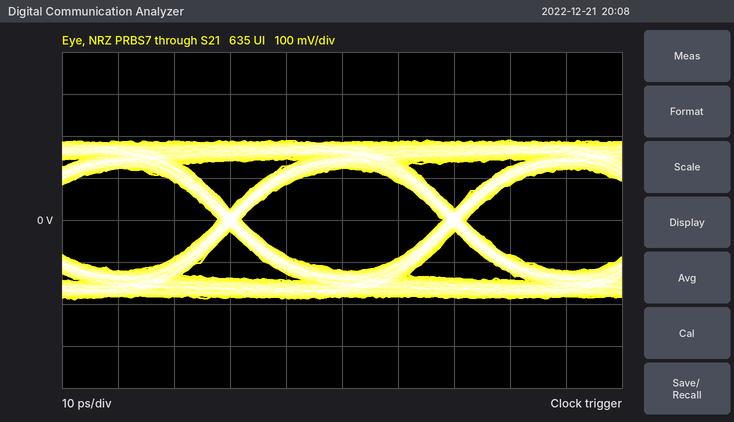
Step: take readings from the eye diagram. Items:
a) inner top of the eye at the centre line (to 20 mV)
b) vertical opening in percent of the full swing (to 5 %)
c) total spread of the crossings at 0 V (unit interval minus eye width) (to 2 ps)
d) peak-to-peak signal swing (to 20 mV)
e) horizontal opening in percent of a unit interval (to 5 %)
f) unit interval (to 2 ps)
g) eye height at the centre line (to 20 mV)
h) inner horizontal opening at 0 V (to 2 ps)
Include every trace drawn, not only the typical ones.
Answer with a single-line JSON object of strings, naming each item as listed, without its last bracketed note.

{"inner top of the eye at the centre line": "120 mV", "vertical opening in percent of the full swing": "65 %", "total spread of the crossings at 0 V (unit interval minus eye width)": "4 ps", "peak-to-peak signal swing": "380 mV", "horizontal opening in percent of a unit interval": "90 %", "unit interval": "40 ps", "eye height at the centre line": "240 mV", "inner horizontal opening at 0 V": "36 ps"}
